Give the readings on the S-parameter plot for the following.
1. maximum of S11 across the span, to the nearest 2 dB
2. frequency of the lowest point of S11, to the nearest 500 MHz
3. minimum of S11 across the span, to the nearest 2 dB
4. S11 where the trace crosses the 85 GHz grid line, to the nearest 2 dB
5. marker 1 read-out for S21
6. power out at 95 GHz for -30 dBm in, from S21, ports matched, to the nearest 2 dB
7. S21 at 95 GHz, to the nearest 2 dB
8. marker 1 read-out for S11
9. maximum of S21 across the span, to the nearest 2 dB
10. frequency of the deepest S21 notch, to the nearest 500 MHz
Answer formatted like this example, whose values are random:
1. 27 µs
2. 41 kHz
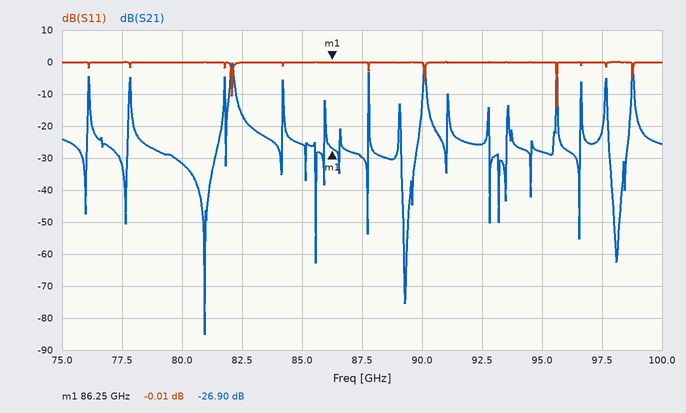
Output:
1. 0 dB
2. 95.5 GHz
3. -14 dB
4. 0 dB
5. -26.90 dB
6. -58 dBm
7. -28 dB
8. -0.01 dB
9. 0 dB
10. 81.0 GHz
